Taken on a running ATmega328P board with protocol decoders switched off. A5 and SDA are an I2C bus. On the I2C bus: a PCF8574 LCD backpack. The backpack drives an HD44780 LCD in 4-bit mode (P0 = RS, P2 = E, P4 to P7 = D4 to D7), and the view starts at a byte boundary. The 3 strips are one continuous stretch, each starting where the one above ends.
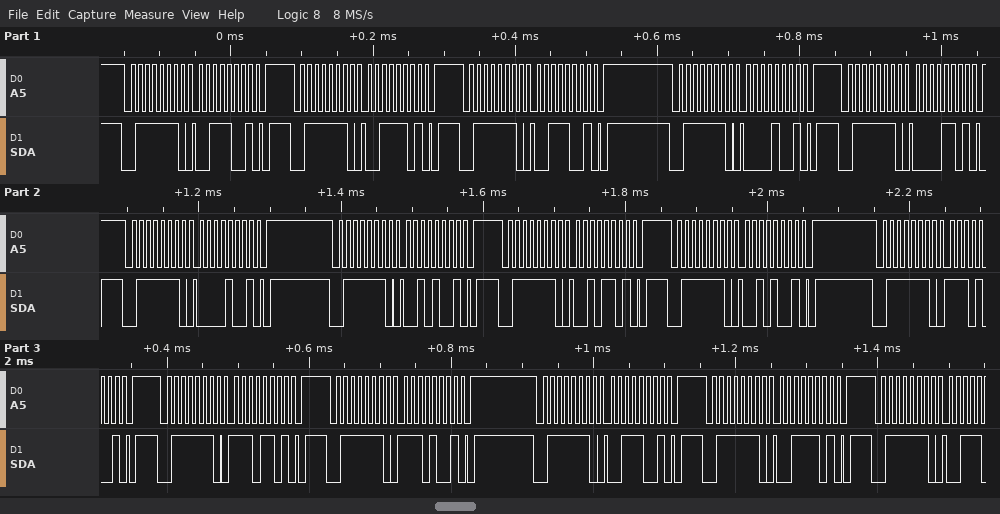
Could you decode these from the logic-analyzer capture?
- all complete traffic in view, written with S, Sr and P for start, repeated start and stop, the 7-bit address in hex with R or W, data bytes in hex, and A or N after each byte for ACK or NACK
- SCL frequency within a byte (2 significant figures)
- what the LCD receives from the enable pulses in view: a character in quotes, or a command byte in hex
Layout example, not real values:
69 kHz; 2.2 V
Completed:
S 3FW A 39 A P S 3FW A 3D A P S 3FW A 39 A P S 3FW A 09 A P S 3FW A 0D A P S 3FW A 09 A P S 3FW A 29 A P S 3FW A 2D A P S 3FW A 29 A P S 3FW A E9 A P S 3FW A ED A P S 3FW A E9 A P S 3FW A 39 A P S 3FW A 3D A P S 3FW A; 100 kHz; '0' '.'
